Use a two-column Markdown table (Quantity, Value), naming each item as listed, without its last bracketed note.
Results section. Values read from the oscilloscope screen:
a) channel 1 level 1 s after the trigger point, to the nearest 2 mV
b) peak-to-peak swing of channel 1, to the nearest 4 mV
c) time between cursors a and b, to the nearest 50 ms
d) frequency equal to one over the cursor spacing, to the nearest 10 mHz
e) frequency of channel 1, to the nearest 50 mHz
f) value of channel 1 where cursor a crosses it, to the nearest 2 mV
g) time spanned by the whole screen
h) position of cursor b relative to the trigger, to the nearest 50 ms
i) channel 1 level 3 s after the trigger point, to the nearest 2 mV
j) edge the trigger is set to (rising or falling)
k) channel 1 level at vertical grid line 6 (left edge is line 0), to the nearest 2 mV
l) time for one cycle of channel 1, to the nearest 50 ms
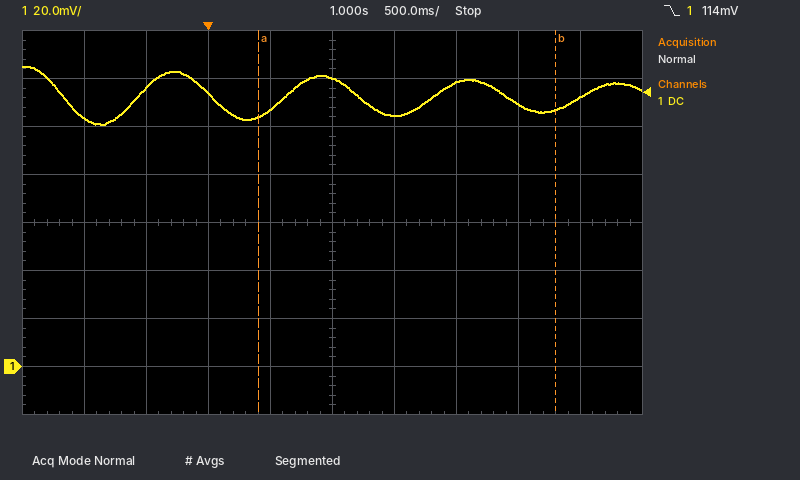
| Quantity | Value |
|---|---|
| channel 1 level 1 s after the trigger point, to the nearest 2 mV | 120 mV |
| peak-to-peak swing of channel 1, to the nearest 4 mV | 24 mV |
| time between cursors a and b, to the nearest 50 ms | 2.40 s |
| frequency equal to one over the cursor spacing, to the nearest 10 mHz | 420 mHz |
| frequency of channel 1, to the nearest 50 mHz | 850 mHz |
| value of channel 1 where cursor a crosses it, to the nearest 2 mV | 104 mV |
| time spanned by the whole screen | 5 s |
| position of cursor b relative to the trigger, to the nearest 50 ms | +2.80 s |
| channel 1 level 3 s after the trigger point, to the nearest 2 mV | 112 mV |
| edge the trigger is set to | falling |
| channel 1 level at vertical grid line 6 (left edge is line 0), to the nearest 2 mV | 104 mV |
| time for one cycle of channel 1, to the nearest 50 ms | 1.20 s |
